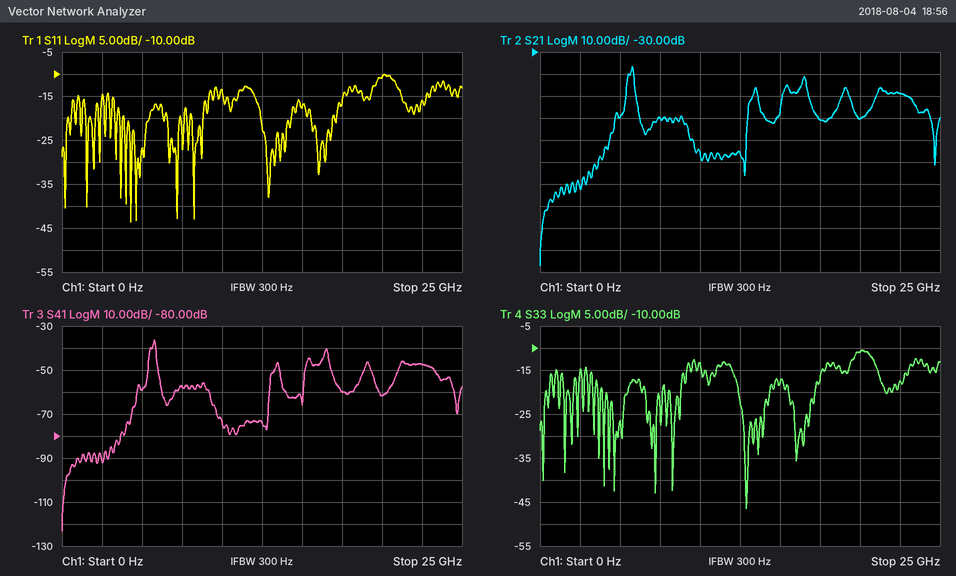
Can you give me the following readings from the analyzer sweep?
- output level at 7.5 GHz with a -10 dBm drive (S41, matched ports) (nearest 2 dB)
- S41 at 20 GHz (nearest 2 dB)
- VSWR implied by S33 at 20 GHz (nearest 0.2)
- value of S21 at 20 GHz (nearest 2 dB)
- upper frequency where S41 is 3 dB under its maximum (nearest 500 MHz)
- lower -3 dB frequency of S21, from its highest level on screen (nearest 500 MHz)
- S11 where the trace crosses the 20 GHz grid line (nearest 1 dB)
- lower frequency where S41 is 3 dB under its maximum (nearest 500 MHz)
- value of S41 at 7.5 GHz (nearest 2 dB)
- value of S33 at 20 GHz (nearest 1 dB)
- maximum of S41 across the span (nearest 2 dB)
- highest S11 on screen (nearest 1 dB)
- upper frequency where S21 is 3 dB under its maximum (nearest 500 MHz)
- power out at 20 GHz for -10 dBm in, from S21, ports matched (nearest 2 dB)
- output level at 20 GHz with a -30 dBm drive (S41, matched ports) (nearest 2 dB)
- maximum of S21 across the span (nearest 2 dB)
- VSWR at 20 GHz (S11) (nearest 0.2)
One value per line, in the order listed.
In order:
-68 dBm
-62 dB
1.8
-60 dB
6.0 GHz
5.5 GHz
-11 dB
5.5 GHz
-58 dB
-11 dB
-36 dB
-10 dB
6.0 GHz
-70 dBm
-92 dBm
-36 dB
1.8
